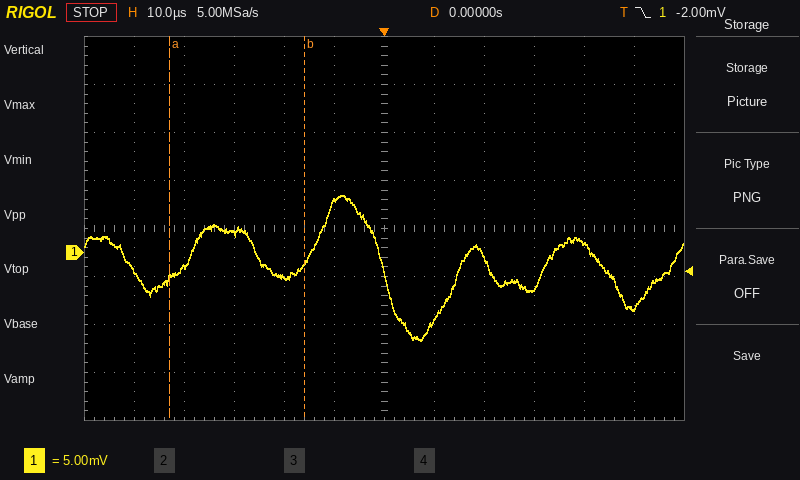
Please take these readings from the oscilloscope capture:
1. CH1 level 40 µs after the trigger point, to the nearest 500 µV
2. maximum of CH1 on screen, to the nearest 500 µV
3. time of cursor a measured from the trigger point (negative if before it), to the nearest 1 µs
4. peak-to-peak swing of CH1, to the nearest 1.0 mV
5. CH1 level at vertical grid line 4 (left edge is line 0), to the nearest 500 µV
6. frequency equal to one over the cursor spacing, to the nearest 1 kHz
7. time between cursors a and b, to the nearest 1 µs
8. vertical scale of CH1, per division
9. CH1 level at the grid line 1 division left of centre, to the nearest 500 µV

1.0 mV
6.0 mV
-43 µs
15.0 mV
-2.5 mV
37 kHz
27 µs
5 mV
5.0 mV
